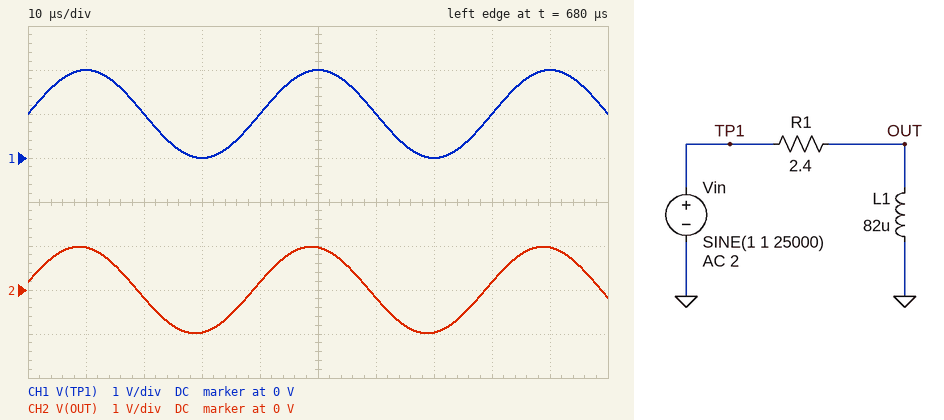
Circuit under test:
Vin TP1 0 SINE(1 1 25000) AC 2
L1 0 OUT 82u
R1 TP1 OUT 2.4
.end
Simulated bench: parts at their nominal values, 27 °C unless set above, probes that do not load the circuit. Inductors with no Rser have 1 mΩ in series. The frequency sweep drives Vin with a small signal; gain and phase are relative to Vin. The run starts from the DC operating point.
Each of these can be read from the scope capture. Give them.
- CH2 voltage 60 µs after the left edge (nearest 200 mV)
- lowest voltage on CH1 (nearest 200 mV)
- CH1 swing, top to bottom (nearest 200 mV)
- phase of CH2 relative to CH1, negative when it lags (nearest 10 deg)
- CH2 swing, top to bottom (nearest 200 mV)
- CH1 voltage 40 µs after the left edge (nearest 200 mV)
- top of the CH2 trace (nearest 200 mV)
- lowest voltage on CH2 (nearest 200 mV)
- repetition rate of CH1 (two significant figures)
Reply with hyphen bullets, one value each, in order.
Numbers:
- -200 mV
- 0 V
- 2.0 V
- 10 deg
- 2.0 V
- 1.0 V
- 1.0 V
- -1.0 V
- 25 kHz
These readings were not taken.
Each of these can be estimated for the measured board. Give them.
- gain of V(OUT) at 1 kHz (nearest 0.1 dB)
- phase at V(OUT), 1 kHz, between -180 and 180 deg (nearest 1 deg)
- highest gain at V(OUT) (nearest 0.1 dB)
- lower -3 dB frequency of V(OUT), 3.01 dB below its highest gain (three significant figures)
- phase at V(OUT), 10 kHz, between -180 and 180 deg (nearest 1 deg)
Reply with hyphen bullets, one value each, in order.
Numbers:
- -13.6 dB
- 78 deg
- 0 dB
- 4.66 kHz
- 25 deg
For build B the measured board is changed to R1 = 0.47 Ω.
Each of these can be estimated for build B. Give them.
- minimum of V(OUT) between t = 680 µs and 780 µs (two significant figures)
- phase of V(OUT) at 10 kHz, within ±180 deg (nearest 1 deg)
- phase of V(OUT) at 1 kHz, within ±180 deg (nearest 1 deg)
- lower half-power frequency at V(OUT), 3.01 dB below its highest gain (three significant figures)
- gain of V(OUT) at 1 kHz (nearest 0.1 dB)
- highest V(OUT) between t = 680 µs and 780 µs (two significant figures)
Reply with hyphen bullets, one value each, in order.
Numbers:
- -1.0 V
- 5 deg
- 42 deg
- 914 Hz
- -2.6 dB
- 1.0 V
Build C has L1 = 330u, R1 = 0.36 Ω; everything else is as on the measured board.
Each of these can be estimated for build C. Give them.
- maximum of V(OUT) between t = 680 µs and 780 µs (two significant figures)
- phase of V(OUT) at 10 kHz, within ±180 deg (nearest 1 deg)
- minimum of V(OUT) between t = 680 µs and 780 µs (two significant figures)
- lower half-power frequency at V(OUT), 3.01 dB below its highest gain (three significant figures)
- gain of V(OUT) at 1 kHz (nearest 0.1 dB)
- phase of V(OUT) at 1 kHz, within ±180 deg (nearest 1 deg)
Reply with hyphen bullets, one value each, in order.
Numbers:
- 1.0 V
- 1 deg
- -1.0 V
- 174 Hz
- -0.1 dB
- 10 deg
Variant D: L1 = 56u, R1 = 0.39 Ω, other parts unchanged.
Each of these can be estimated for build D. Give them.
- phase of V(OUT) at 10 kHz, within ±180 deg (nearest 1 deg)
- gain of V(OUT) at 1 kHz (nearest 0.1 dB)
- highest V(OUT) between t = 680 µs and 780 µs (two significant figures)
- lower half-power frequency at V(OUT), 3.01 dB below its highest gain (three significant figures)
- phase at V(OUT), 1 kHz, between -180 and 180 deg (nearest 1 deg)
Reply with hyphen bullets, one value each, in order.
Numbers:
- 6 deg
- -3.5 dB
- 1.0 V
- 1.11 kHz
- 48 deg
